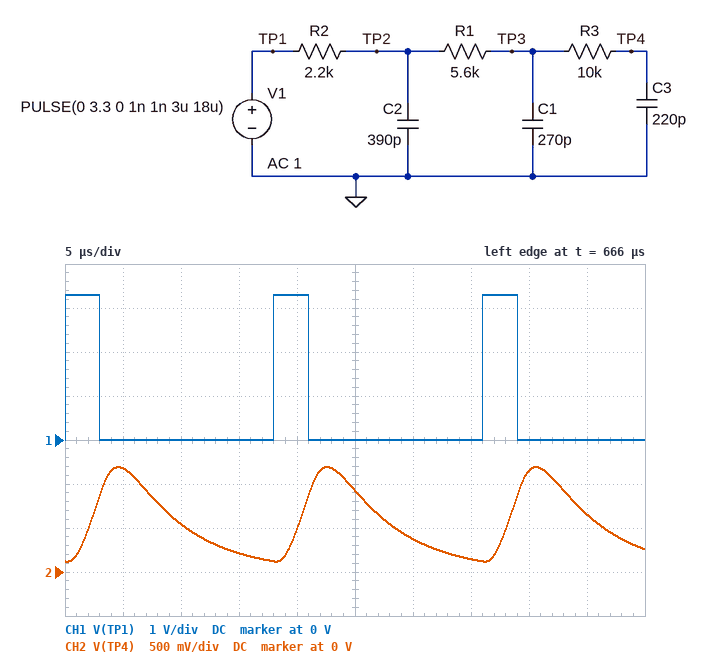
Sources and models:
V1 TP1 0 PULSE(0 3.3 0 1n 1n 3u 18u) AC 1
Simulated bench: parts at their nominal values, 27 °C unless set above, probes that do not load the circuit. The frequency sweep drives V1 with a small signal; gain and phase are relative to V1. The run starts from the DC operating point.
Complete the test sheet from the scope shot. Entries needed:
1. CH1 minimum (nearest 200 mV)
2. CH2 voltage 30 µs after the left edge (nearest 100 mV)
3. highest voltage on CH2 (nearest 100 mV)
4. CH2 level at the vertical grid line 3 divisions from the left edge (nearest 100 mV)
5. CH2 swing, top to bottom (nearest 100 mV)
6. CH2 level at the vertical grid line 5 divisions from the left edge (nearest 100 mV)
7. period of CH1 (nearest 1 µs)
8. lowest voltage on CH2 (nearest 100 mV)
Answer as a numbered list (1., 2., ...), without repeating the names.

1. 0 V
2. 400 mV
3. 1.2 V
4. 200 mV
5. 1.1 V
6. 900 mV
7. 18 µs
8. 100 mV
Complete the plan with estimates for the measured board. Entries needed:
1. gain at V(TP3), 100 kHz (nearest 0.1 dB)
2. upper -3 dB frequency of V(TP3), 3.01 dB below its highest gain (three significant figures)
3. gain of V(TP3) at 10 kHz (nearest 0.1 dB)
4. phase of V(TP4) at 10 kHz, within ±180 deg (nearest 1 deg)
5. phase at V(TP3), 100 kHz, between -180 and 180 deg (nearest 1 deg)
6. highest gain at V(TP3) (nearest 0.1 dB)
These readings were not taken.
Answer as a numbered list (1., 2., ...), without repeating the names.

1. -8.2 dB
2. 34.1 kHz
3. -0.4 dB
4. -24 deg
5. -71 deg
6. 0 dB
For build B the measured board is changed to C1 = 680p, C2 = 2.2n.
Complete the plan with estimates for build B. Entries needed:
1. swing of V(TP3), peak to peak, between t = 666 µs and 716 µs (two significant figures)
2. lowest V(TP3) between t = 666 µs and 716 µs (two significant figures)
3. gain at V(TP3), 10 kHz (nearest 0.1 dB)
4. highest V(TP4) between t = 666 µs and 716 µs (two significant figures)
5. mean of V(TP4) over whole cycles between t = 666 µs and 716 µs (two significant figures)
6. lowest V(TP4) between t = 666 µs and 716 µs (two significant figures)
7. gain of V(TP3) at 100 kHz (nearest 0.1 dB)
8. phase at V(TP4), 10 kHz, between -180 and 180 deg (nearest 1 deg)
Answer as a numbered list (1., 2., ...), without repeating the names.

1. 530 mV
2. 280 mV
3. -1.5 dB
4. 730 mV
5. 550 mV
6. 340 mV
7. -20.2 dB
8. -47 deg
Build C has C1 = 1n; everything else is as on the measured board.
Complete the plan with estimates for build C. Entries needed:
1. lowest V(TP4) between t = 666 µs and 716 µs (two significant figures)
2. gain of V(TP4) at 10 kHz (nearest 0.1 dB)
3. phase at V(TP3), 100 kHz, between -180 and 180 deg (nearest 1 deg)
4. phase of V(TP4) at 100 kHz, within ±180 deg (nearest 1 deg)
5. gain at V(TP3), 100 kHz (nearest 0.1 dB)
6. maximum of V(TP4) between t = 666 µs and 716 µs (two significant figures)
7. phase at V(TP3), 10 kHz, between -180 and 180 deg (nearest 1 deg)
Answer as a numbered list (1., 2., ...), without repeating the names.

1. 290 mV
2. -1.6 dB
3. -95 deg
4. -149 deg
5. -15.6 dB
6. 820 mV
7. -33 deg
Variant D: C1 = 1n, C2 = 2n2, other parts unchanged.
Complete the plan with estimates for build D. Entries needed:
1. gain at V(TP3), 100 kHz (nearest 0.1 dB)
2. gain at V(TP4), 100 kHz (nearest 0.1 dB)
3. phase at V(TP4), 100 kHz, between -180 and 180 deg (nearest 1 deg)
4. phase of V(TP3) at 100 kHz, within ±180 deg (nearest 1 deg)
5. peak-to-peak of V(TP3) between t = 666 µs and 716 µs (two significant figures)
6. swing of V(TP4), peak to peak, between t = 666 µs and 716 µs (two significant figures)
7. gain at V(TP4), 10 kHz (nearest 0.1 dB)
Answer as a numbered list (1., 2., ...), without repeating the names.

1. -22.8 dB
2. -27.4 dB
3. 169 deg
4. -137 deg
5. 410 mV
6. 310 mV
7. -2.1 dB
